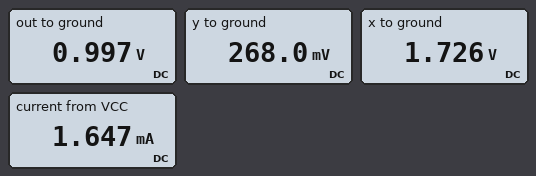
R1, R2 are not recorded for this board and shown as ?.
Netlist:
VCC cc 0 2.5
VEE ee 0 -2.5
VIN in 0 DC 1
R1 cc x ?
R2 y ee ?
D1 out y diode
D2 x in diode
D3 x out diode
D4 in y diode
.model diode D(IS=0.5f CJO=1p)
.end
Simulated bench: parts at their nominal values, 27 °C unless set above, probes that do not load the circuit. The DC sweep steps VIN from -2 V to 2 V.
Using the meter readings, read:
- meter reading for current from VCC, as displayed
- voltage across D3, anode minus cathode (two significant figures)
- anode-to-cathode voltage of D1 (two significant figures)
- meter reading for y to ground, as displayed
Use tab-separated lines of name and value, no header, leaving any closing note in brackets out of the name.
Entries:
meter reading for current from VCC, as displayed	1.647 mA
voltage across D3, anode minus cathode	730 mV
anode-to-cathode voltage of D1	730 mV
meter reading for y to ground, as displayed	268.0 mV
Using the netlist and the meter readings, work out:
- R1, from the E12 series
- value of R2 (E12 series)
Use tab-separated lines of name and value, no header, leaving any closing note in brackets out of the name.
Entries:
R1, from the E12 series	470 Ω
value of R2	1.5 kΩ
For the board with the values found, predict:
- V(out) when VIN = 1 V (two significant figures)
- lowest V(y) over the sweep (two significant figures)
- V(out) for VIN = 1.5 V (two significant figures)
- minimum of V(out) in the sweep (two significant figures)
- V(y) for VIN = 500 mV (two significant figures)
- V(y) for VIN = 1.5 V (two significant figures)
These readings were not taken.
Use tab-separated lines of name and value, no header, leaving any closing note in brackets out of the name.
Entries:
V(out) when VIN = 1 V	1.0 V
lowest V(y) over the sweep	-2.5 V
V(out) for VIN = 1.5 V	1.5 V
minimum of V(out) in the sweep	-1.8 V
V(y) for VIN = 500 mV	-220 mV
V(y) for VIN = 1.5 V	750 mV
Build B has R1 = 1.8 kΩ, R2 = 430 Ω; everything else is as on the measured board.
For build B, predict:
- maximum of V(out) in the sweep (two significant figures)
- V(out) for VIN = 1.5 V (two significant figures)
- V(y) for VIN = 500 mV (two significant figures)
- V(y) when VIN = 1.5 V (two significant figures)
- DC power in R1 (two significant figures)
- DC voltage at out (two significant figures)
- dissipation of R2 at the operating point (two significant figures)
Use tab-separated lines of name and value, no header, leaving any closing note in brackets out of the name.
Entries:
maximum of V(out) in the sweep	1.8 V
V(out) for VIN = 1.5 V	1.4 V
V(y) for VIN = 500 mV	-270 mV
V(y) when VIN = 1.5 V	720 mV
DC power in R1	410 µW
DC voltage at out	930 mV
dissipation of R2 at the operating point	17 mW
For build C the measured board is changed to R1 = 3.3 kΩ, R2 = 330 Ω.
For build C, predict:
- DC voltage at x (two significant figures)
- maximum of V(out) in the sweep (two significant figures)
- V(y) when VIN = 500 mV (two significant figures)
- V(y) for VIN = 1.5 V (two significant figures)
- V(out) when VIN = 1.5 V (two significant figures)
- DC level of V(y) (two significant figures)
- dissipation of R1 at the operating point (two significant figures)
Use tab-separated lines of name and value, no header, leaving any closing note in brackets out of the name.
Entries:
DC voltage at x	1.6 V
maximum of V(out) in the sweep	1.8 V
V(y) when VIN = 500 mV	-280 mV
V(y) for VIN = 1.5 V	710 mV
V(out) when VIN = 1.5 V	1.4 V
DC level of V(y)	210 mV
dissipation of R1 at the operating point	240 µW
